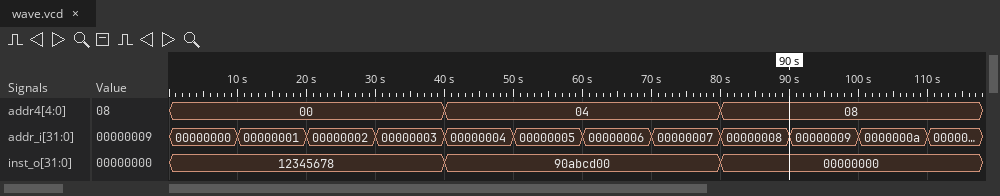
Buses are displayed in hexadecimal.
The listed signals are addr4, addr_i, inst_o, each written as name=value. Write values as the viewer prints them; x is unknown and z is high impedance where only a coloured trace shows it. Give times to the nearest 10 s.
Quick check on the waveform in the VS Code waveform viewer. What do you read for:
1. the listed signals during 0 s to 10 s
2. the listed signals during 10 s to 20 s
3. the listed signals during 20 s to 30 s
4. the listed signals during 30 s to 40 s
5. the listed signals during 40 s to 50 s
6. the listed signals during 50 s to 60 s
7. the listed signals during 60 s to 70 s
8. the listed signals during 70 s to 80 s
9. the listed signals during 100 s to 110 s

addr4=00, addr_i=00000000, inst_o=12345678
addr4=00, addr_i=00000001, inst_o=12345678
addr4=00, addr_i=00000002, inst_o=12345678
addr4=00, addr_i=00000003, inst_o=12345678
addr4=04, addr_i=00000004, inst_o=90abcd00
addr4=04, addr_i=00000005, inst_o=90abcd00
addr4=04, addr_i=00000006, inst_o=90abcd00
addr4=04, addr_i=00000007, inst_o=90abcd00
addr4=08, addr_i=0000000a, inst_o=00000000
